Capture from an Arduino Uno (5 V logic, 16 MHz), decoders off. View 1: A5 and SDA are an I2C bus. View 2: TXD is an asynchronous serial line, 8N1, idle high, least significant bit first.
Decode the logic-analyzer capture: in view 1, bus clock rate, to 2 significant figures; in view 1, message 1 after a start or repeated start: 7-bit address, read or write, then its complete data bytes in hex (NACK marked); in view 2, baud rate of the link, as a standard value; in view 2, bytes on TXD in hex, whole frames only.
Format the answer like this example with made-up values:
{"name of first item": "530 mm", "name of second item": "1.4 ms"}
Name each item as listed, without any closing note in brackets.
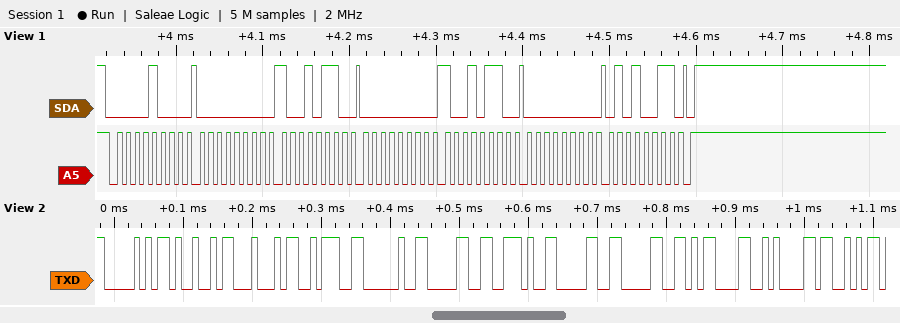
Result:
{"in view 1, bus clock rate, to 2 significant figures": "100 kHz", "in view 1, message 1 after a start or repeated start: 7-bit address, read or write, then its complete data bytes in hex": "0x04 write: 00 96 00 96 00 53", "in view 2, baud rate of the link, as a standard value": "115200 baud", "in view 2, bytes on TXD in hex, whole frames only": "50 49 44 3A 20 30 2E 30 30 0D 0A 53"}
